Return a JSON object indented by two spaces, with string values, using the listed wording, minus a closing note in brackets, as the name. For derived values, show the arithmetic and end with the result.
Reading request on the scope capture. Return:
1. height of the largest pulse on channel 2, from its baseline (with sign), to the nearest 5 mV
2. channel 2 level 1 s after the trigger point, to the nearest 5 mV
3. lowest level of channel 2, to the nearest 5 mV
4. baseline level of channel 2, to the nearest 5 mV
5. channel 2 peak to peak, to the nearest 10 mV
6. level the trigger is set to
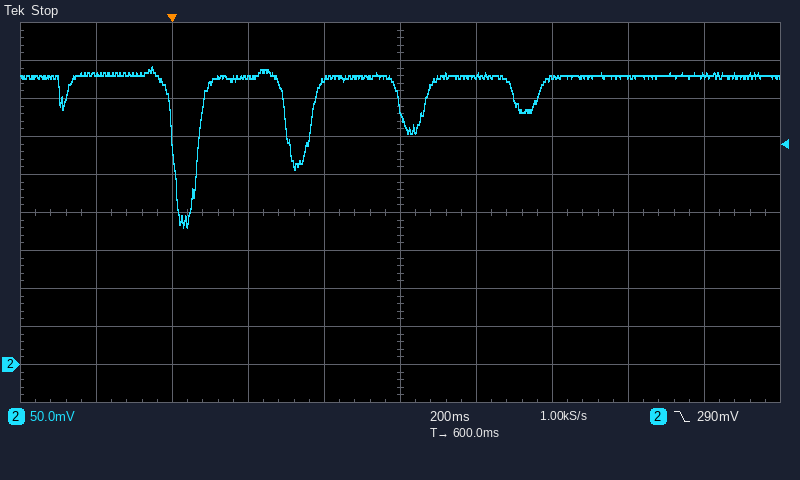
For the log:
{
  "height of the largest pulse on channel 2, from its baseline (with sign), to the nearest 5 mV": "180 mV − (380 mV) = -200 mV",
  "channel 2 level 1 s after the trigger point, to the nearest 5 mV": "375 mV",
  "lowest level of channel 2, to the nearest 5 mV": "180 mV",
  "baseline level of channel 2, to the nearest 5 mV": "380 mV",
  "channel 2 peak to peak, to the nearest 10 mV": "210 mV",
  "level the trigger is set to": "290 mV"
}
